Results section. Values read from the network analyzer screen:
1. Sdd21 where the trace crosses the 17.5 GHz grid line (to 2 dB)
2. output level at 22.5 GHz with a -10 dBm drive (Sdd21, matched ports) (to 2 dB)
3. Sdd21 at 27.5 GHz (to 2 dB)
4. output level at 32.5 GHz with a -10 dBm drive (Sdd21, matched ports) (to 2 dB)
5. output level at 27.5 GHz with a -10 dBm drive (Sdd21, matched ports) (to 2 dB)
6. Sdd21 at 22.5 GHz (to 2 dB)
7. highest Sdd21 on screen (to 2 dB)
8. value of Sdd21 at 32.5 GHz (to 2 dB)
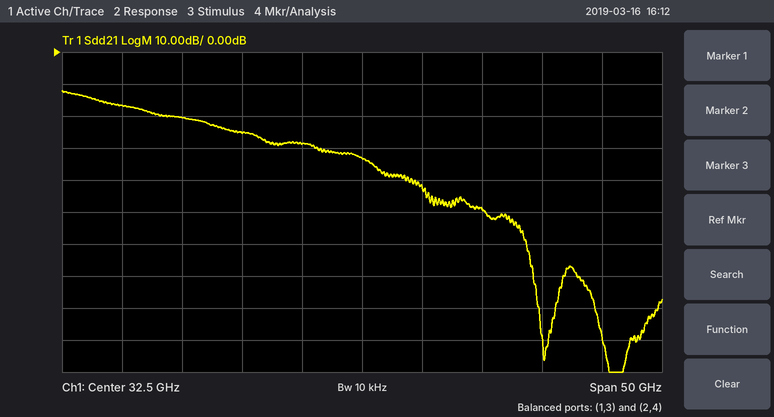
-20 dB
-36 dBm
-28 dB
-44 dBm
-38 dBm
-26 dB
-12 dB
-34 dB
